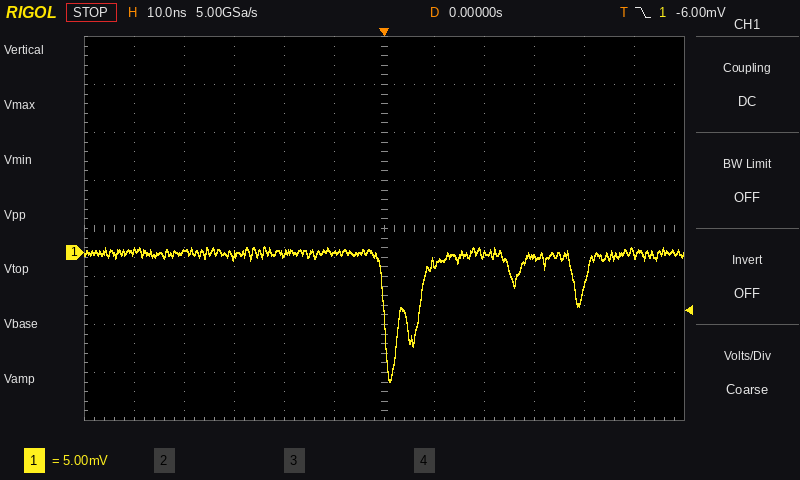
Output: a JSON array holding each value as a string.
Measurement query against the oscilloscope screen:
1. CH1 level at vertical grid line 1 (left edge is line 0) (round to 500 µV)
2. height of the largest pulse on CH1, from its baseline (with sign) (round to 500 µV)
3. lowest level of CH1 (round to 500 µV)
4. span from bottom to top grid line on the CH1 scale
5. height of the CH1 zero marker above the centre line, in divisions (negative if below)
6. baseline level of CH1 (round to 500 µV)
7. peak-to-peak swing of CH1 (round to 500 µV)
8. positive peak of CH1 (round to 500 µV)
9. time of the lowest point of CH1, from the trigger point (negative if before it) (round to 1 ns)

["0.0 mV", "-13.5 mV", "-13.5 mV", "40 mV", "-0.5 div", "0.0 mV", "14.0 mV", "500 µV", "+1 ns"]
